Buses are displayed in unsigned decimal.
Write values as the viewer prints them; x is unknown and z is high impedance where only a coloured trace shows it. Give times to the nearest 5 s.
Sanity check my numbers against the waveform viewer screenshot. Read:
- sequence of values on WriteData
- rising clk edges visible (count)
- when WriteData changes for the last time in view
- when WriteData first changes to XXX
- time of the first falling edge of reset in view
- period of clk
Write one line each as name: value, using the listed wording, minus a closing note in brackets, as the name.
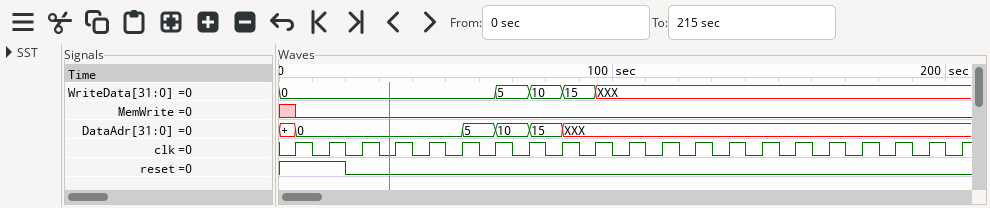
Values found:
sequence of values on WriteData: 0, 5, 10, 15, XXX
rising clk edges visible: 21
when WriteData changes for the last time in view: 95 s
when WriteData first changes to XXX: 95 s
time of the first falling edge of reset in view: 20 s
period of clk: 10 s
